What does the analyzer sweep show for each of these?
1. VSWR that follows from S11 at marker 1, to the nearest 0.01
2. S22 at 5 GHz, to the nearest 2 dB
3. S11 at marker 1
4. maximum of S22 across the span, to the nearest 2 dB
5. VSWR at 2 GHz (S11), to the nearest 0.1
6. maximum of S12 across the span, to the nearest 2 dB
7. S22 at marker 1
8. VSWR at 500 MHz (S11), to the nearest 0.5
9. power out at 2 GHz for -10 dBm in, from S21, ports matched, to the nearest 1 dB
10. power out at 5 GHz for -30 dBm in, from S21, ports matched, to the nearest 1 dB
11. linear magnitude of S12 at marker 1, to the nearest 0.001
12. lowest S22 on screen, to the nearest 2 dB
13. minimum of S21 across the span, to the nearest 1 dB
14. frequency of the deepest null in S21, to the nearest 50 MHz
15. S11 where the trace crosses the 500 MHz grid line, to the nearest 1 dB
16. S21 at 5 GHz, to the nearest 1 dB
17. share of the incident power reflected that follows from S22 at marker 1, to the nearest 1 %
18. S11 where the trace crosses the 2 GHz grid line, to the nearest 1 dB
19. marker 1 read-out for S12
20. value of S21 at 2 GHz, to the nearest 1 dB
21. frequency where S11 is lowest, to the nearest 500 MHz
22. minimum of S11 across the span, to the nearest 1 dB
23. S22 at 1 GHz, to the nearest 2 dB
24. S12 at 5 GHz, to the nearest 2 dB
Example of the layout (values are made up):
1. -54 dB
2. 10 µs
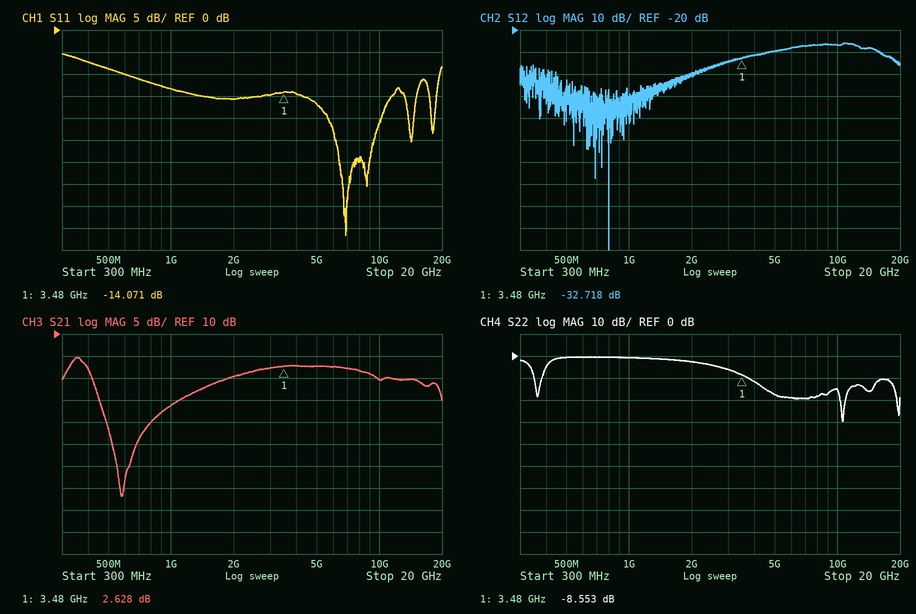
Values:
1. 1.49
2. -18 dB
3. -14.071 dB
4. 0 dB
5. 1.4
6. -26 dB
7. -8.553 dB
8. 2.0
9. -10 dBm
10. -27 dBm
11. 0.023
12. -30 dB
13. -27 dB
14. 600 MHz
15. -9 dB
16. 3 dB
17. 14 %
18. -16 dB
19. -32.718 dB
20. 0 dB
21. 7.0 GHz
22. -47 dB
23. 0 dB
24. -30 dB
